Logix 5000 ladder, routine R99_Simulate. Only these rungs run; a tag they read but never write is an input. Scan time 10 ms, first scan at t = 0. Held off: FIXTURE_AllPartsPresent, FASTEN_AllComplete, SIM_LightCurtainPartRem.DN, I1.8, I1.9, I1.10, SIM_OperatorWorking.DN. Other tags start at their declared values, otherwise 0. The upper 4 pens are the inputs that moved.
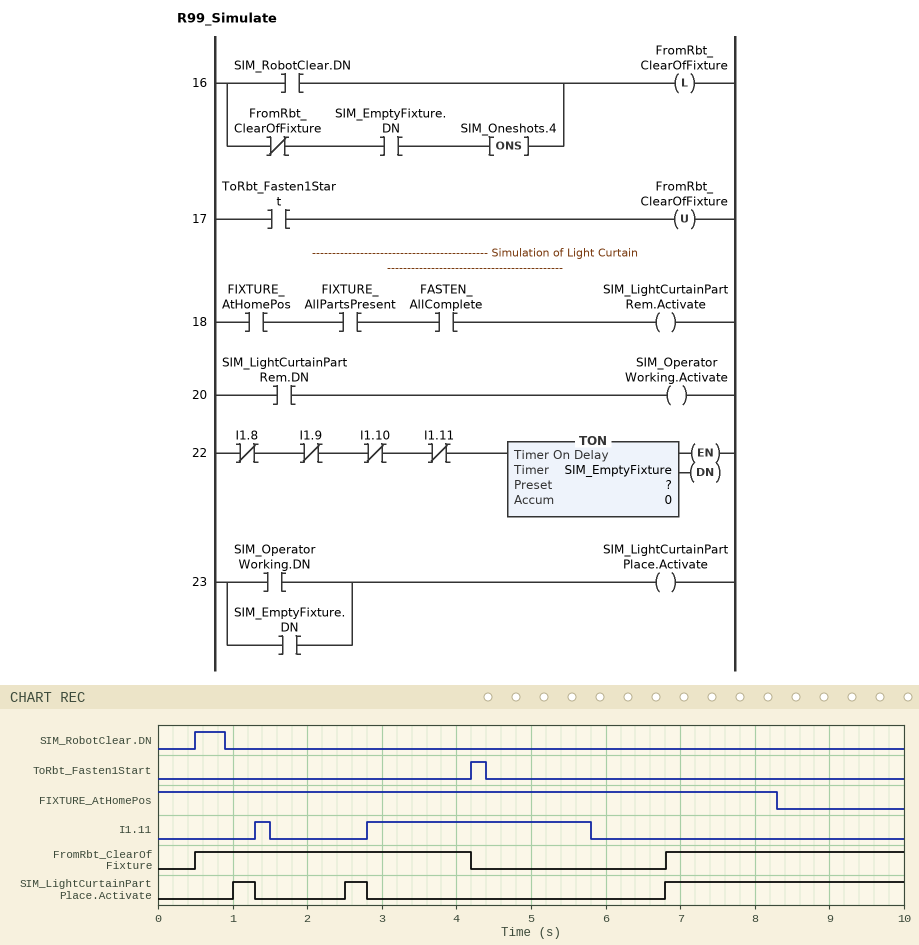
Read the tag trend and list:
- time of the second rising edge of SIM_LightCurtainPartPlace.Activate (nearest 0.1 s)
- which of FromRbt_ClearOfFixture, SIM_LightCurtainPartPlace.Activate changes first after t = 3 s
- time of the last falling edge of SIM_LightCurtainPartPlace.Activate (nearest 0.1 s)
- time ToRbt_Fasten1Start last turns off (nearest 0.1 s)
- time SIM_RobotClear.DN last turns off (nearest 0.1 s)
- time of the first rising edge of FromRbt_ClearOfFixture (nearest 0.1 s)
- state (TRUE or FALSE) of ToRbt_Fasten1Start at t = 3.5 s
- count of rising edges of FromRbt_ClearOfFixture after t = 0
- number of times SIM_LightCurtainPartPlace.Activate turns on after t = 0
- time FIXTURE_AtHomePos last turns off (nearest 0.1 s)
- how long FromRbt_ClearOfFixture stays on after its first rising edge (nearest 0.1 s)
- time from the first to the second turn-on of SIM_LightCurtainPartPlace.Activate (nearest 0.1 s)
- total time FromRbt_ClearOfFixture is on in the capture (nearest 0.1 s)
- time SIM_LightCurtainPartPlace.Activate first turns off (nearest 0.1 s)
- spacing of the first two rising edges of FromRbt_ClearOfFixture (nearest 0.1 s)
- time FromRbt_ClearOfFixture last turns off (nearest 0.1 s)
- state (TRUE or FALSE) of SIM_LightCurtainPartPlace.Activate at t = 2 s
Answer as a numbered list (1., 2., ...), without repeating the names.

1. 2.5 s
2. FromRbt_ClearOfFixture
3. 2.8 s
4. 4.4 s
5. 0.9 s
6. 0.5 s
7. FALSE
8. 2
9. 3
10. 8.3 s
11. 3.7 s
12. 1.5 s
13. 6.9 s
14. 1.3 s
15. 6.3 s
16. 4.2 s
17. FALSE
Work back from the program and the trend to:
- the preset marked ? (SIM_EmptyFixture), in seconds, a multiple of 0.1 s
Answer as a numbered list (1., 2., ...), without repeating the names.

1. 1.0 s
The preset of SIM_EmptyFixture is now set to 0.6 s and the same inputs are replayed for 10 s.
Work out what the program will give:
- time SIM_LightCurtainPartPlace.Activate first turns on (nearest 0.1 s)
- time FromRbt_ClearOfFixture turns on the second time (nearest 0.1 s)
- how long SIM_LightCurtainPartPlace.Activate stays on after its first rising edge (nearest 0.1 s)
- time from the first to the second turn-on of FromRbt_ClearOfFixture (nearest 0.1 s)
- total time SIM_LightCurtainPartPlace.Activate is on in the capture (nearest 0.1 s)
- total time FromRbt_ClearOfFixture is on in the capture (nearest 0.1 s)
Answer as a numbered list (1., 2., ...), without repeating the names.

1. 0.6 s
2. 6.4 s
3. 0.7 s
4. 5.9 s
5. 5.0 s
6. 7.3 s
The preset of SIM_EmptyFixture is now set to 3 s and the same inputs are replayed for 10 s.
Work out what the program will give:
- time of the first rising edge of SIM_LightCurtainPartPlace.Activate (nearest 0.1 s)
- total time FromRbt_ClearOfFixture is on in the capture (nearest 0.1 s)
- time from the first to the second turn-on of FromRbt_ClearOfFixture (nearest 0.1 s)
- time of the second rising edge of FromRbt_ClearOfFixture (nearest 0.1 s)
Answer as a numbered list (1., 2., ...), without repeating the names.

1. 8.8 s
2. 4.9 s
3. 8.3 s
4. 8.8 s
